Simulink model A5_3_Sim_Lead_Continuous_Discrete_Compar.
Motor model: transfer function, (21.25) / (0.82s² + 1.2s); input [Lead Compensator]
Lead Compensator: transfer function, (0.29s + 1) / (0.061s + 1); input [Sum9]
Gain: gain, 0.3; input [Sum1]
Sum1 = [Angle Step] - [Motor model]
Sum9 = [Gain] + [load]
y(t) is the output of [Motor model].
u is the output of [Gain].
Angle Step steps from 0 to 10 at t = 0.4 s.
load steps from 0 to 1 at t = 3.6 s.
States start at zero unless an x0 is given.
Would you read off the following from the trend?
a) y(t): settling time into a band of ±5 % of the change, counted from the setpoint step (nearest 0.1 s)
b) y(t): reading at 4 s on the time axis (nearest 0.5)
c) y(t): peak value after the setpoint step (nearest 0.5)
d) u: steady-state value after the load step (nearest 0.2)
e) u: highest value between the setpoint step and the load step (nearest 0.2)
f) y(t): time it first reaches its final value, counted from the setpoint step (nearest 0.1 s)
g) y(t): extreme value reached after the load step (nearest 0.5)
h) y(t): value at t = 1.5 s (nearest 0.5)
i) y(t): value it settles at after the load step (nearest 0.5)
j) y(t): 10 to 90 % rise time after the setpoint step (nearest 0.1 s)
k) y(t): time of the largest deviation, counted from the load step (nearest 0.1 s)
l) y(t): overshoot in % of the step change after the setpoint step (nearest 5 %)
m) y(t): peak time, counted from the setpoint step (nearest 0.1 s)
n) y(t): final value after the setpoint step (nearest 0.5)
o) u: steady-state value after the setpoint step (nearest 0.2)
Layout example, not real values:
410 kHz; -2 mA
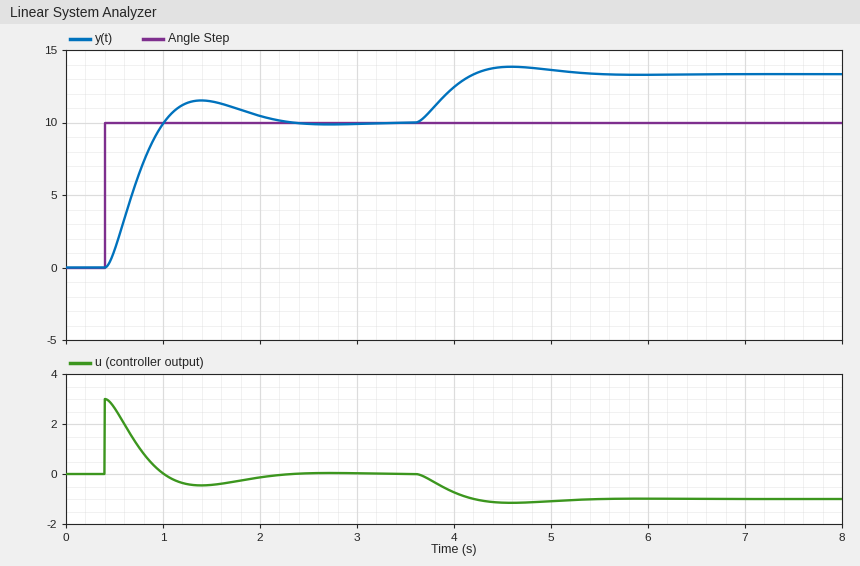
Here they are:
1.6 s; 12.5; 11.5; -1.0; 3.0; 0.6 s; 14.0; 11.5; 13.5; 0.4 s; 1.0 s; 15 %; 1.0 s; 10.0; 0.0
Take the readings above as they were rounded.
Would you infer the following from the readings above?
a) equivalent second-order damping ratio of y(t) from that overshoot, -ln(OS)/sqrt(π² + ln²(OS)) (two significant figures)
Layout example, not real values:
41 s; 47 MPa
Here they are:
0.52
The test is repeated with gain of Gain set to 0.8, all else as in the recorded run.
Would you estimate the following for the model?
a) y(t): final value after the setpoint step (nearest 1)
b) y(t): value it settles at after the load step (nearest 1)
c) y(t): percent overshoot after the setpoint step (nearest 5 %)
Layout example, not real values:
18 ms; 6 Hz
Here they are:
10; 11; 20 %
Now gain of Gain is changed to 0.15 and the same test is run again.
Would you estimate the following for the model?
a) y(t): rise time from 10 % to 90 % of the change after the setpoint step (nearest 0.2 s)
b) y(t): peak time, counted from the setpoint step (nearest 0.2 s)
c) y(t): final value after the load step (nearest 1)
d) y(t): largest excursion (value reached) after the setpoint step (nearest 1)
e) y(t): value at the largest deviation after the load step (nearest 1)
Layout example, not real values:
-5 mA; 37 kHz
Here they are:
0.8 s; 1.6 s; 17; 11; 17
